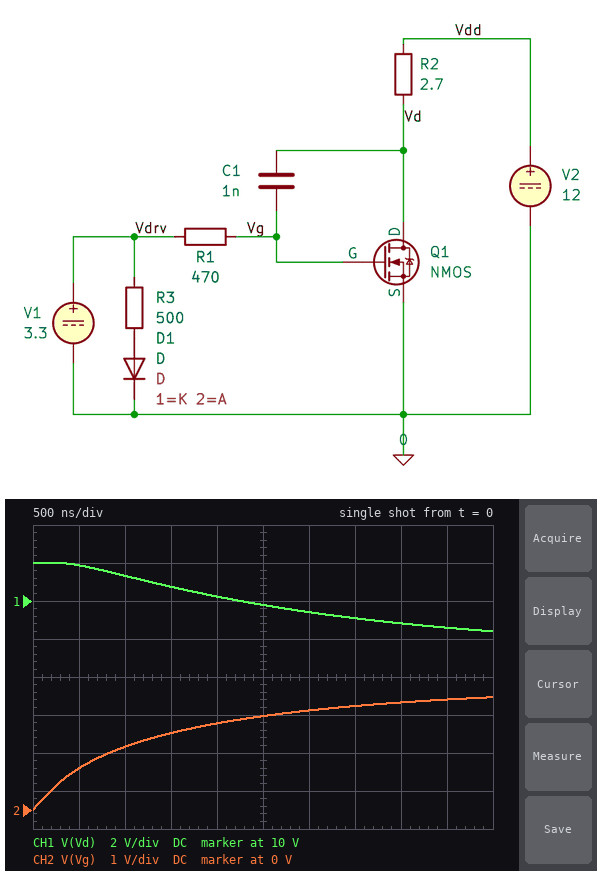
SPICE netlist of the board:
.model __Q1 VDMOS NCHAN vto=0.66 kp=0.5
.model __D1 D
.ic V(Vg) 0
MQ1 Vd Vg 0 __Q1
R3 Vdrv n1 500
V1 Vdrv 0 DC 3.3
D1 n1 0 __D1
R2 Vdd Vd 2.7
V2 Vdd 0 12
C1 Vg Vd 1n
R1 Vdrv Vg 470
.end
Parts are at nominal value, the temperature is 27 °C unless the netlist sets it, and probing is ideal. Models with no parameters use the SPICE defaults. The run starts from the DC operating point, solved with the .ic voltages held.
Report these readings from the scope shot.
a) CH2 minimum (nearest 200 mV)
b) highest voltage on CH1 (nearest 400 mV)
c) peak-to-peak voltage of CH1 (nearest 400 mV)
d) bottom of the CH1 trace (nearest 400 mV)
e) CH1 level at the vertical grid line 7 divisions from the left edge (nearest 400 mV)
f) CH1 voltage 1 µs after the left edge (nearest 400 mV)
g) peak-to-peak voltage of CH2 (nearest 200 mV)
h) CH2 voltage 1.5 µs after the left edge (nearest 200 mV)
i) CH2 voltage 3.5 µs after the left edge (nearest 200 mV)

0 V
12.0 V
3.6 V
8.4 V
9.2 V
11.2 V
3.0 V
2.0 V
2.8 V
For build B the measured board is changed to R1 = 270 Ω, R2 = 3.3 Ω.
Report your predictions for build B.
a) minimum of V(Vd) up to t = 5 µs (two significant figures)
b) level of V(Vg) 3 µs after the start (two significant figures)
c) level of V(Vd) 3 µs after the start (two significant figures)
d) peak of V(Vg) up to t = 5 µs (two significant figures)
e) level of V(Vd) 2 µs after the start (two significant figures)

6.8 V
2.9 V
7.7 V
3.2 V
8.7 V
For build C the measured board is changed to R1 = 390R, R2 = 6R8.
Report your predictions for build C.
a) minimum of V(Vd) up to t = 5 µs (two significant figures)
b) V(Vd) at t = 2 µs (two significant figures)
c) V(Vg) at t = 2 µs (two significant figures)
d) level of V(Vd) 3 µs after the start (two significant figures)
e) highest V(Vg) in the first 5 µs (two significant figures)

4.6 V
8.4 V
2.1 V
6.8 V
2.7 V
